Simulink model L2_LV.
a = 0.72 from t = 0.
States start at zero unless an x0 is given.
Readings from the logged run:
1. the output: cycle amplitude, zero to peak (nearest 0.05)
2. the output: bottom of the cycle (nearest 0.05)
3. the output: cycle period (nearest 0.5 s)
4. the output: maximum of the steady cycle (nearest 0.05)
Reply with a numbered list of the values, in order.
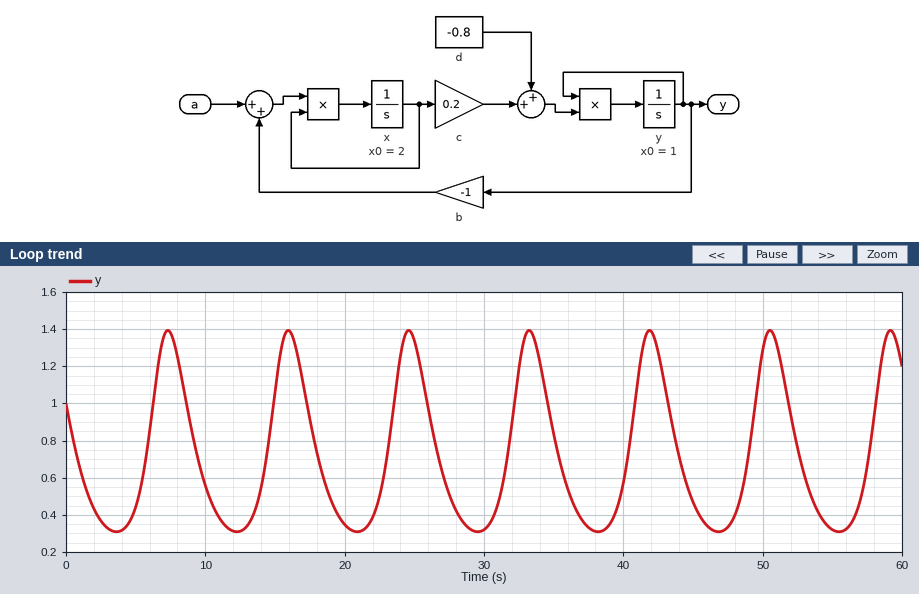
1. 0.55
2. 0.30
3. 8.5 s
4. 1.40
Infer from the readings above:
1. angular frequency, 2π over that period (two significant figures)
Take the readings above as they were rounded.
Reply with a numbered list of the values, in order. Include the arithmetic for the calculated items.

1. 2π / 8.5 = 0.74 rad/s
